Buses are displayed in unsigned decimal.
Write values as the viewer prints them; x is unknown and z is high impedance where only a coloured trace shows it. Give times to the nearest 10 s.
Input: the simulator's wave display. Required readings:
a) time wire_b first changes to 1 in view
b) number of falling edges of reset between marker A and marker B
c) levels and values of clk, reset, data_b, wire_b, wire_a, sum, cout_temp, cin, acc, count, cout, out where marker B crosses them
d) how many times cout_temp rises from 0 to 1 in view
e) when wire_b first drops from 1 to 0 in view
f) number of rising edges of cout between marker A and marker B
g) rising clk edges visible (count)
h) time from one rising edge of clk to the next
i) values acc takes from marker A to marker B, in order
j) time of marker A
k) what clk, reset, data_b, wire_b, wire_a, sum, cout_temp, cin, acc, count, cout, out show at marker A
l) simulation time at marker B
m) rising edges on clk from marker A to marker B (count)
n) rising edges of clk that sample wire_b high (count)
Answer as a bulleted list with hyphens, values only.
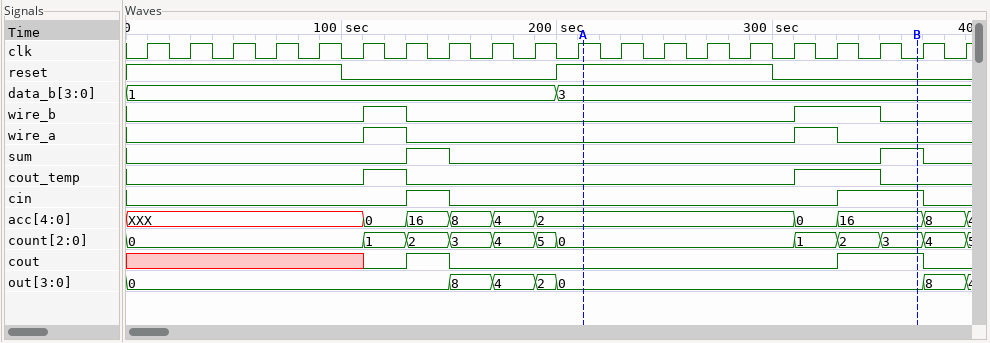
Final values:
- 110 s
- 1
- clk=0, reset=0, data_b=3, wire_b=0, wire_a=0, sum=1, cout_temp=0, cin=1, acc=16, count=3, cout=1, out=0
- 2
- 130 s
- 1
- 20
- 20 s
- 2, 0, 16
- 210 s
- clk=1, reset=1, data_b=3, wire_b=0, wire_a=0, sum=0, cout_temp=0, cin=0, acc=2, count=0, cout=0, out=0
- 370 s
- 7
- 3
